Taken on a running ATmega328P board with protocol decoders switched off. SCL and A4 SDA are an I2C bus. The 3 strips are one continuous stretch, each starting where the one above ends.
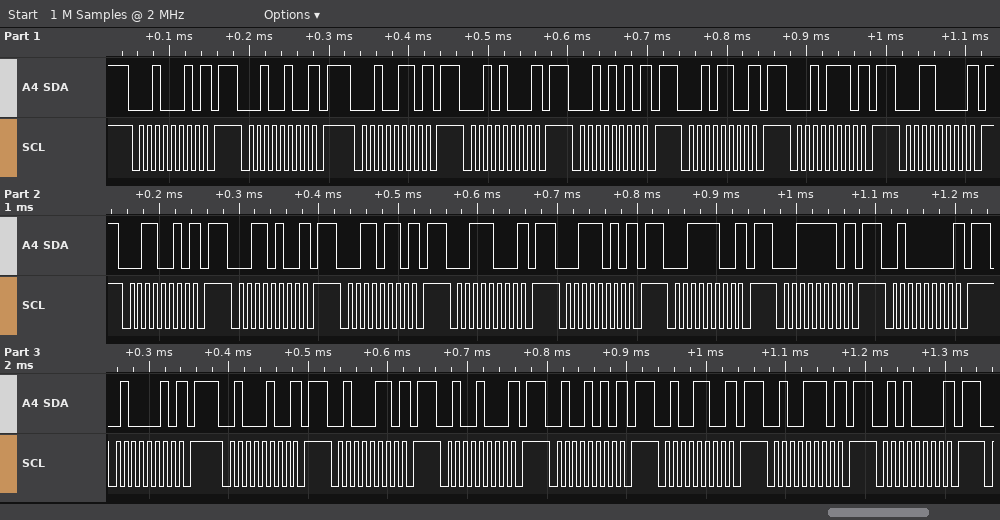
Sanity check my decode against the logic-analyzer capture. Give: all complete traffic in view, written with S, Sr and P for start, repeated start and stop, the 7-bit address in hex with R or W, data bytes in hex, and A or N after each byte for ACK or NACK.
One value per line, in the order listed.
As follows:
S 11W N P S 12W N P S 13W N P S 14W N P S 15W N P S 16W N P S 17W N P S 18W N P S 19W N P S 1AW N P S 1BW N P S 1CW N P S 1DW N P S 1EW N P S 1FW N P S 20W N P S 21W N P S 22W N P S 23W N P S 24W N P S 25W N P S 26W N P S 27W N P S 28W N P
